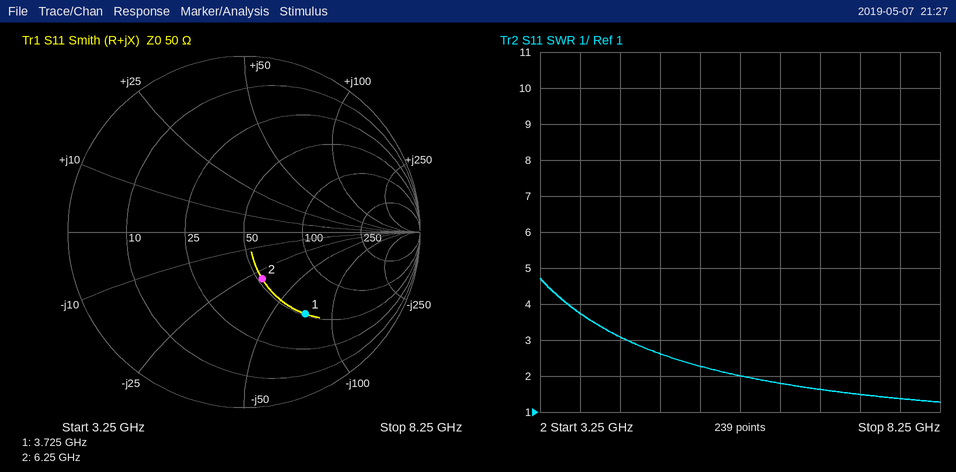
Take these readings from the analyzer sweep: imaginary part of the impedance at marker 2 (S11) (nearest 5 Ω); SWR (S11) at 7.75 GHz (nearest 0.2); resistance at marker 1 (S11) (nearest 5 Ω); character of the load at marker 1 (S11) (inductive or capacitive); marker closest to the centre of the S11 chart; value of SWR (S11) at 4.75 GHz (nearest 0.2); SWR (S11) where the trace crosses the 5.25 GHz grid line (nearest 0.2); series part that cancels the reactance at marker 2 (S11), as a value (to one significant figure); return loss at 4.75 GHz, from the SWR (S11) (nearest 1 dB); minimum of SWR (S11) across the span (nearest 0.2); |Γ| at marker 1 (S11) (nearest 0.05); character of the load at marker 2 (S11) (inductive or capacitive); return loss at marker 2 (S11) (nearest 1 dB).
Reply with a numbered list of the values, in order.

1. -30 Ω
2. 1.4
3. 50 Ω
4. capacitive
5. marker 2
6. 2.6
7. 2.2
8. 800 pH
9. 7 dB
10. 1.2
11. 0.60
12. capacitive
13. 11 dB
